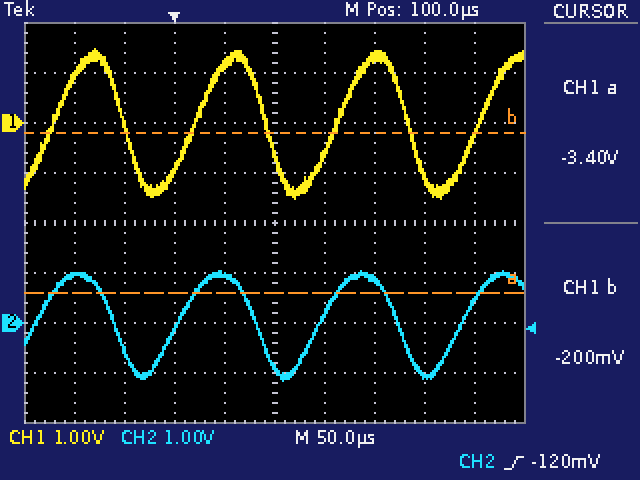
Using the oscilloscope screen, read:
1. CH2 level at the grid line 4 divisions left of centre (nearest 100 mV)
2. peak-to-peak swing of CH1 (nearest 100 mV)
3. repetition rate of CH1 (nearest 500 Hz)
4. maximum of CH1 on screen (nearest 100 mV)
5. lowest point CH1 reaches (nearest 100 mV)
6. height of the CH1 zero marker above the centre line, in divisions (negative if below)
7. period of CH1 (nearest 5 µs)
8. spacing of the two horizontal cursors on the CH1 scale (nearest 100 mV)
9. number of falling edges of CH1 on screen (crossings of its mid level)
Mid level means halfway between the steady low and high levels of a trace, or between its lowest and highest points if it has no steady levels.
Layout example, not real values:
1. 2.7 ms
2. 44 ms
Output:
1. 900 mV
2. 3.0 V
3. 7.0 kHz
4. 1.5 V
5. -1.5 V
6. +2.0 div
7. 140 µs
8. 3.2 V
9. 3
